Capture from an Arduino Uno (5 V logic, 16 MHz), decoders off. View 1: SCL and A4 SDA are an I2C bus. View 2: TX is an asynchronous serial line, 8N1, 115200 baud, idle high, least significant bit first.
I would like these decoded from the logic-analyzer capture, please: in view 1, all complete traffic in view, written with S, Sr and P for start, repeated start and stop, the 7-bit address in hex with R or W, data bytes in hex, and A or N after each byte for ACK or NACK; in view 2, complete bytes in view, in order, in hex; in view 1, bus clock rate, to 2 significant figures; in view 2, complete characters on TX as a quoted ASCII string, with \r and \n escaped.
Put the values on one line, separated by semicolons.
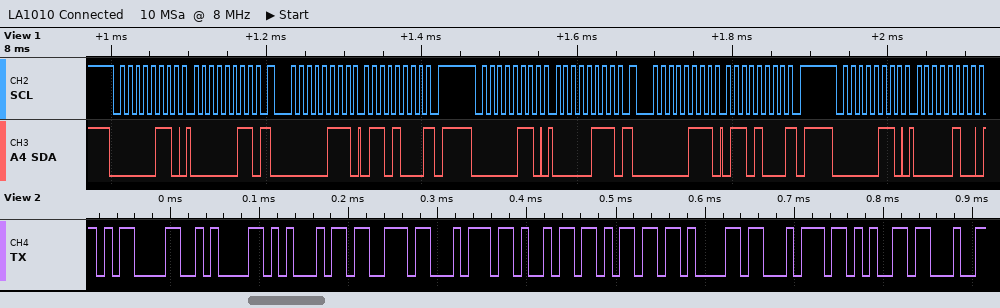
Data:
S 03W A 03 A Sr 03R A 68 N P S 03W A 07 A Sr 03R A 68 N P S 03W A 04 A; 0x0D 0x0A 0x45 0x73 0x74 0x69 0x6D 0x61 0x74 0x65; 100 kHz; "\r\nEstimate"
